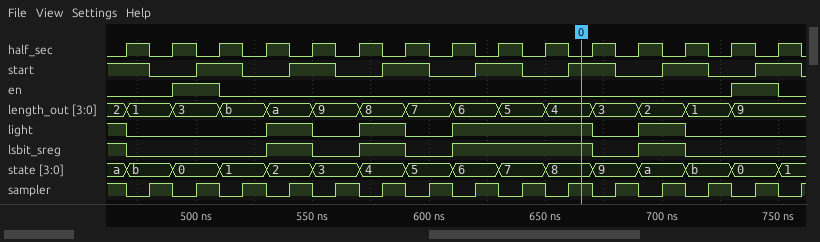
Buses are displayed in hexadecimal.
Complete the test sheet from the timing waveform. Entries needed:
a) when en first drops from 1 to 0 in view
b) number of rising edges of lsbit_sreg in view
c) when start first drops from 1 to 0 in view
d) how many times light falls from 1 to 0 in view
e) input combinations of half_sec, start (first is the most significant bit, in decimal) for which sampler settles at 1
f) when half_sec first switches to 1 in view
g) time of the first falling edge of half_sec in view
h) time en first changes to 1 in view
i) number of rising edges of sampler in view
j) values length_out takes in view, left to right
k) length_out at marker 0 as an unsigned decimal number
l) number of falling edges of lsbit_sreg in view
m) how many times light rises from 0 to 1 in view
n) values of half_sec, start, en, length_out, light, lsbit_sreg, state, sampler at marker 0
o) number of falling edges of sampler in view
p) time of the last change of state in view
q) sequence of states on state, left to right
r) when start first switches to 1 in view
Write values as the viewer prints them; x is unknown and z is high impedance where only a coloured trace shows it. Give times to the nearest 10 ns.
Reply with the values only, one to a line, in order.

510 ns
4
480 ns
5
0, 1
470 ns
480 ns
490 ns
15
2, 1, 3, b, a, 9, 8, 7, 6, 5, 4, 3, 2, 1, 9
4
5
4
half_sec=0, start=1, en=0, length_out=4, light=1, lsbit_sreg=1, state=8, sampler=1
15
750 ns
a, b, 0, 1, 2, 3, 4, 5, 6, 7, 8, 9, a, b, 0, 1
500 ns
